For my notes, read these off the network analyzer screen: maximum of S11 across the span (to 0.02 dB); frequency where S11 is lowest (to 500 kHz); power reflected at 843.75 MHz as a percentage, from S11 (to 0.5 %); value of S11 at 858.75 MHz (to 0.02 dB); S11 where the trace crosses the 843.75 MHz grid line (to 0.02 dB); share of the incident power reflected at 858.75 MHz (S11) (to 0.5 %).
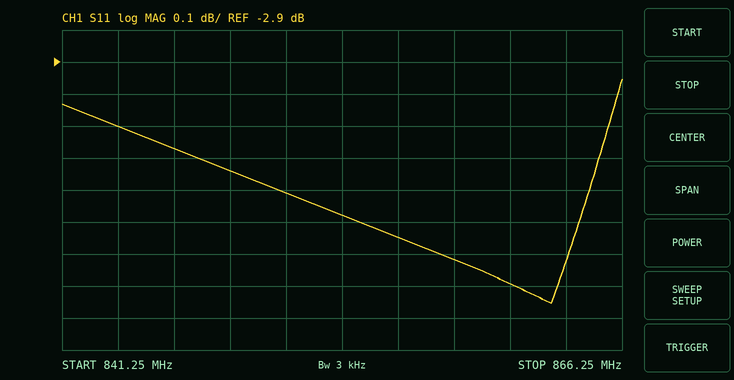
-2.96 dB
863.0 MHz
49.0 %
-3.52 dB
-3.10 dB
44.5 %
